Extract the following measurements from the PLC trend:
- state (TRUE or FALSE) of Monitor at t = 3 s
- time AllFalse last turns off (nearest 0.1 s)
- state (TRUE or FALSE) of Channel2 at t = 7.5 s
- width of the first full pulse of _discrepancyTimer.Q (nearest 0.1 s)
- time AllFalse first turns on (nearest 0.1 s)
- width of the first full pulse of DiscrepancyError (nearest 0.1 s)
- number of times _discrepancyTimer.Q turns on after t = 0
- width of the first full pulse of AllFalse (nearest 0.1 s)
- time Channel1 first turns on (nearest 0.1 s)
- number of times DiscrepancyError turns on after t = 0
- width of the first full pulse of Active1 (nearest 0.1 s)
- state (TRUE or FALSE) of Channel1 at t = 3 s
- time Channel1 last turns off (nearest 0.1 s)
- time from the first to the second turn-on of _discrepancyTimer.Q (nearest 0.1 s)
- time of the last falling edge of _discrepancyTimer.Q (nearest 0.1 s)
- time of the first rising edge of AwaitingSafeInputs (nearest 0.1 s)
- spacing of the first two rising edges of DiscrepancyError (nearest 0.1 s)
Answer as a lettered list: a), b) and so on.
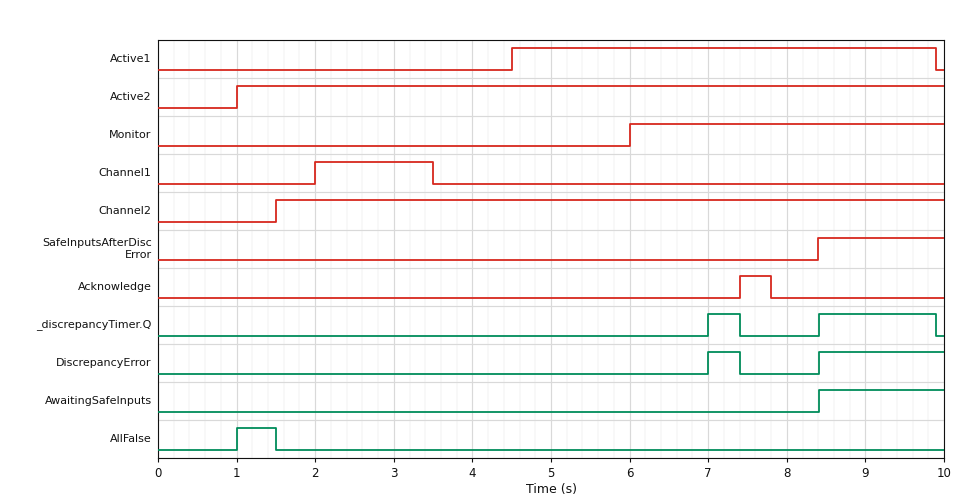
a) FALSE
b) 1.5 s
c) TRUE
d) 0.4 s
e) 1.0 s
f) 0.4 s
g) 2
h) 0.5 s
i) 2.0 s
j) 2
k) 5.4 s
l) TRUE
m) 3.5 s
n) 1.4 s
o) 9.9 s
p) 8.4 s
q) 1.4 s
